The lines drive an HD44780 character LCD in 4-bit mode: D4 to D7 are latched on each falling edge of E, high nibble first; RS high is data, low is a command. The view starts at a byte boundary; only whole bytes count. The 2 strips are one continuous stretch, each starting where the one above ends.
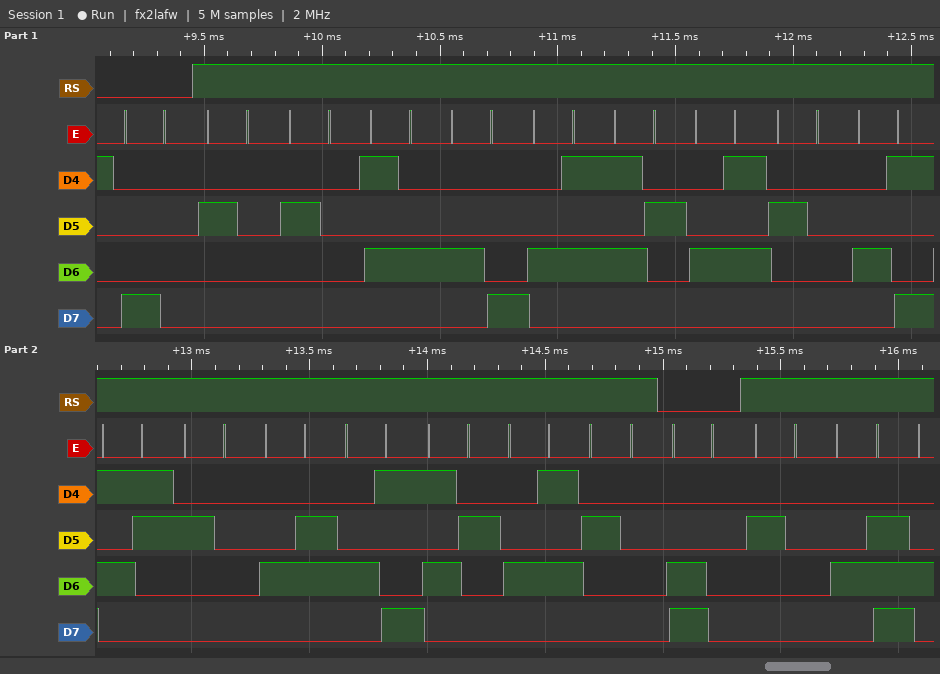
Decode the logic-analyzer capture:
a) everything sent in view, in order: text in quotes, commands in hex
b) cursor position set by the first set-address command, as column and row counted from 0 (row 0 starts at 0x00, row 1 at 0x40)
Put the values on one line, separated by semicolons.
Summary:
0x80 "  THERE IS FIRE " 0xC0 " N"; column 0, row 0
